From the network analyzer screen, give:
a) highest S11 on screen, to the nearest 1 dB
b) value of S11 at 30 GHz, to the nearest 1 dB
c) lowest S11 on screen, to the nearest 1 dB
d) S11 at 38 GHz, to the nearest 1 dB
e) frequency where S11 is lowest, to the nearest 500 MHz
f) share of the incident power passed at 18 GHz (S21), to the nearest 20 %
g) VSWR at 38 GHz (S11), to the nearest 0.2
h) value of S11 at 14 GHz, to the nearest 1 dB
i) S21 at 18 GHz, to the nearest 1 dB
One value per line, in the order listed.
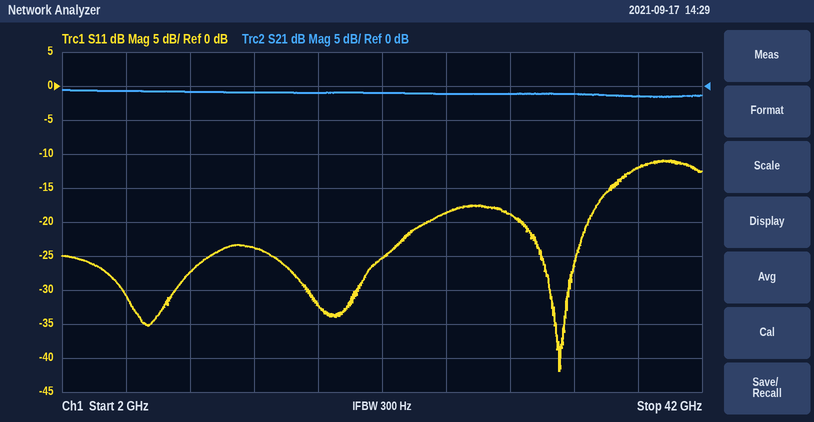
-11 dB
-19 dB
-42 dB
-12 dB
33.0 GHz
80 %
1.6
-24 dB
-1 dB
